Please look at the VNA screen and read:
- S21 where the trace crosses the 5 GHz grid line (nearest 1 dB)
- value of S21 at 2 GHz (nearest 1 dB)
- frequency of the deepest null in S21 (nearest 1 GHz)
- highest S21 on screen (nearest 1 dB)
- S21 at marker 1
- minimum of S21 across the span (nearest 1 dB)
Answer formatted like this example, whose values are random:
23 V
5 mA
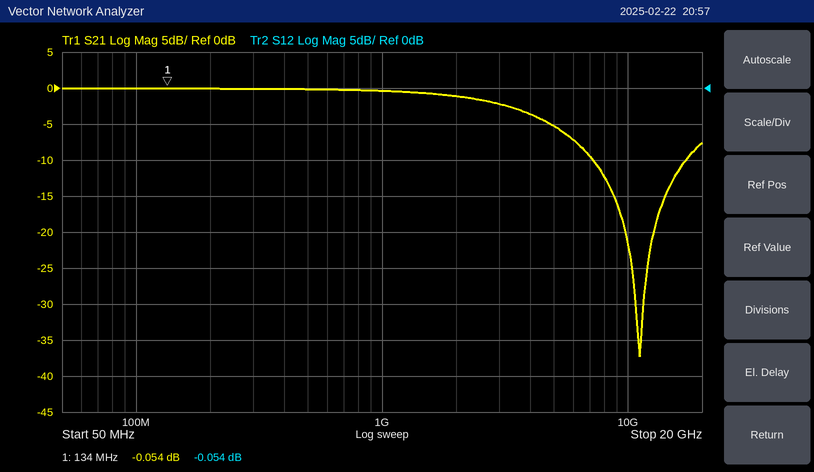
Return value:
-5 dB
-1 dB
11 GHz
0 dB
-0.054 dB
-37 dB
